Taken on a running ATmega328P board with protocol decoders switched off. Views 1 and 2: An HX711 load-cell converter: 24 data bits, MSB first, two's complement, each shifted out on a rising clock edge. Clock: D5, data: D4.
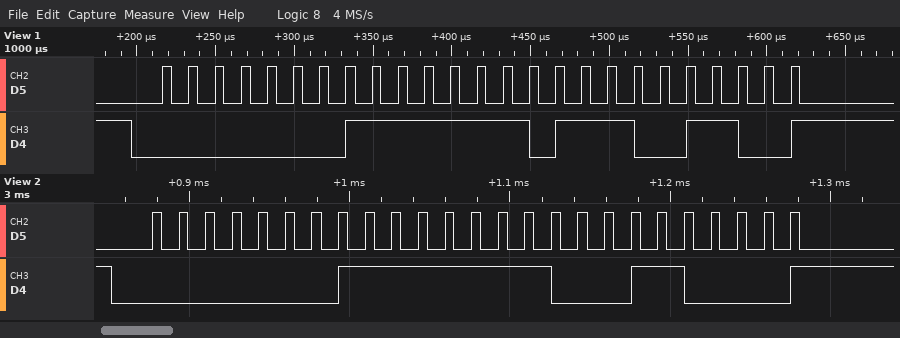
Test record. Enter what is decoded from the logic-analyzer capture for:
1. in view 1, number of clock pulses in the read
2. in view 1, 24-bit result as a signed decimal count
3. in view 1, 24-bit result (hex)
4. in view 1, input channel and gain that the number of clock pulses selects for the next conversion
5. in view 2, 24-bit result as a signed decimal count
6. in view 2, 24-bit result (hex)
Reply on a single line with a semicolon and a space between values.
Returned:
25; 130508; 0x01FDCC; channel A, gain 128; 130608; 0x01FE30
